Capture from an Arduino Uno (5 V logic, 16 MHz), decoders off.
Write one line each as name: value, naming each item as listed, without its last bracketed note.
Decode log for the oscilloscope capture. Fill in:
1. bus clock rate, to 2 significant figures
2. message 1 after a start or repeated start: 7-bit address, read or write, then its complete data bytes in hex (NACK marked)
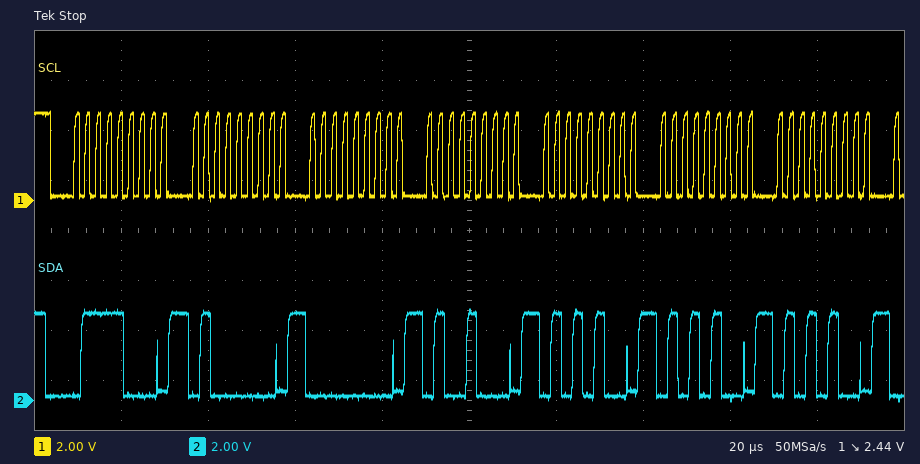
bus clock rate, to 2 significant figures: 400 kHz
message 1 after a start or repeated start: 7-bit address, read or write, then its complete data bytes in hex: 0x3C write: 40 00 48 54 54 54
